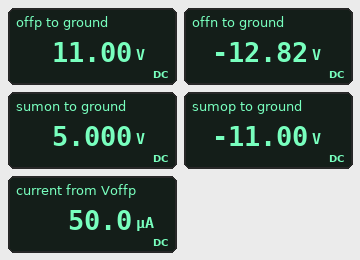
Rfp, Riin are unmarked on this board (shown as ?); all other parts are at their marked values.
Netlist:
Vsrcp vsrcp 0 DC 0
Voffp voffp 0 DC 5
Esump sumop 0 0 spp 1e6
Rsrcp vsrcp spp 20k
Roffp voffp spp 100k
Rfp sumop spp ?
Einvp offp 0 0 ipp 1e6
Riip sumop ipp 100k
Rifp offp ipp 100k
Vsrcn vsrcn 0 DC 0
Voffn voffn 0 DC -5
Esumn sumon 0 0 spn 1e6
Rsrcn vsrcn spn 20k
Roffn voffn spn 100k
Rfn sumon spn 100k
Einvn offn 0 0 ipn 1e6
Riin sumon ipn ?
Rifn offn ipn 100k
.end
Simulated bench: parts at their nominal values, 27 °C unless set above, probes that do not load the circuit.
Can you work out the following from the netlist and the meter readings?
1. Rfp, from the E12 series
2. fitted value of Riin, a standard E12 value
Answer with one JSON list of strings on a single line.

["220 kΩ", "39 kΩ"]
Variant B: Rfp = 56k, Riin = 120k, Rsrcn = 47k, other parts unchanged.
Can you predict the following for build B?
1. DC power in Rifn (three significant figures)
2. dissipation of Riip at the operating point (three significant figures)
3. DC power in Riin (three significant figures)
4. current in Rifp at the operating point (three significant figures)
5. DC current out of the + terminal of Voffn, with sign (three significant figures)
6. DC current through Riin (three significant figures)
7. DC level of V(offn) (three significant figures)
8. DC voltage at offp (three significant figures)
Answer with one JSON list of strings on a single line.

["174 µW", "78.4 µW", "208 µW", "28.0 µA", "-50.0 µA", "41.7 µA", "-4.17 V", "2.80 V"]
